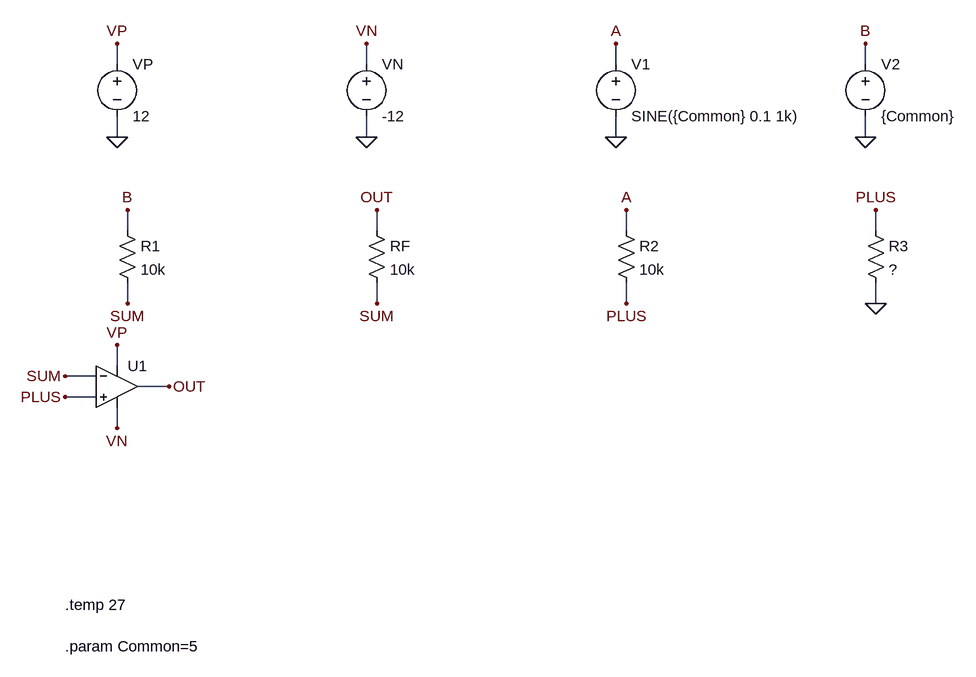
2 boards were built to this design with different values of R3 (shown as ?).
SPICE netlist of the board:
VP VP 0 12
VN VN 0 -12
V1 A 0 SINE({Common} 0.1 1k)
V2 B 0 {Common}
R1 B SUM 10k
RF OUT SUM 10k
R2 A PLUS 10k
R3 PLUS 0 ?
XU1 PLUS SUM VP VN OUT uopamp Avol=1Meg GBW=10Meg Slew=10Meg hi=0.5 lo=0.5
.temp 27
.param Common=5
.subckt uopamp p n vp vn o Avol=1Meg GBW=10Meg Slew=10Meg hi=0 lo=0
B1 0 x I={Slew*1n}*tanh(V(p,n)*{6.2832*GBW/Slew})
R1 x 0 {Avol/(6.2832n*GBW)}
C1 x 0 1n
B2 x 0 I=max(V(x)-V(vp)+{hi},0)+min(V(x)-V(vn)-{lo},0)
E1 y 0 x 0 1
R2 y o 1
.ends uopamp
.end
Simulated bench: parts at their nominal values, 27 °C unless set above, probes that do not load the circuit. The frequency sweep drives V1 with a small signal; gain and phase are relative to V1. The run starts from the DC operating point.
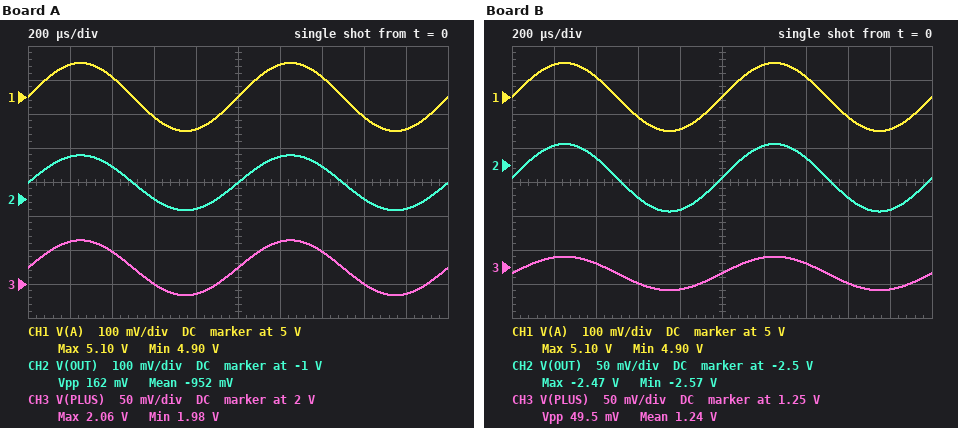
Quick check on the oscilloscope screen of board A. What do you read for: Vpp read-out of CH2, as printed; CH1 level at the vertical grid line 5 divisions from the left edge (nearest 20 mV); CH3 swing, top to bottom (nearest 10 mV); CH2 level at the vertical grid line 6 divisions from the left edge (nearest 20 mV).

162 mV
5.00 V
80 mV
-880 mV
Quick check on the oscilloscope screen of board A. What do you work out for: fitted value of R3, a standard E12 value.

6.8 kΩ
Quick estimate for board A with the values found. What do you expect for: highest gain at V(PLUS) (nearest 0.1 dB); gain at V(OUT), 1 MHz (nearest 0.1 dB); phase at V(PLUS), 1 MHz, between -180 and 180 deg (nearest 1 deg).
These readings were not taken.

-7.9 dB
-2.0 dB
0 deg
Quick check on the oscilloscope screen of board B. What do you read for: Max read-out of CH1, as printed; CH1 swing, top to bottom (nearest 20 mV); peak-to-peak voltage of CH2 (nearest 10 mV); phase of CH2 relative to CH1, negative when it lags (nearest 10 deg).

5.10 V
200 mV
100 mV
0 deg
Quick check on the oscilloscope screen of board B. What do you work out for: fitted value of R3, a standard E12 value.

3.3 kΩ
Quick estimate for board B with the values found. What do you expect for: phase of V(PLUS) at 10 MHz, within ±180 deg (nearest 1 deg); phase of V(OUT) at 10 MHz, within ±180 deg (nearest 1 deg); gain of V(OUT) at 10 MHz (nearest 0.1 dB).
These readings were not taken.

0 deg
-63 deg
-13.1 dB
